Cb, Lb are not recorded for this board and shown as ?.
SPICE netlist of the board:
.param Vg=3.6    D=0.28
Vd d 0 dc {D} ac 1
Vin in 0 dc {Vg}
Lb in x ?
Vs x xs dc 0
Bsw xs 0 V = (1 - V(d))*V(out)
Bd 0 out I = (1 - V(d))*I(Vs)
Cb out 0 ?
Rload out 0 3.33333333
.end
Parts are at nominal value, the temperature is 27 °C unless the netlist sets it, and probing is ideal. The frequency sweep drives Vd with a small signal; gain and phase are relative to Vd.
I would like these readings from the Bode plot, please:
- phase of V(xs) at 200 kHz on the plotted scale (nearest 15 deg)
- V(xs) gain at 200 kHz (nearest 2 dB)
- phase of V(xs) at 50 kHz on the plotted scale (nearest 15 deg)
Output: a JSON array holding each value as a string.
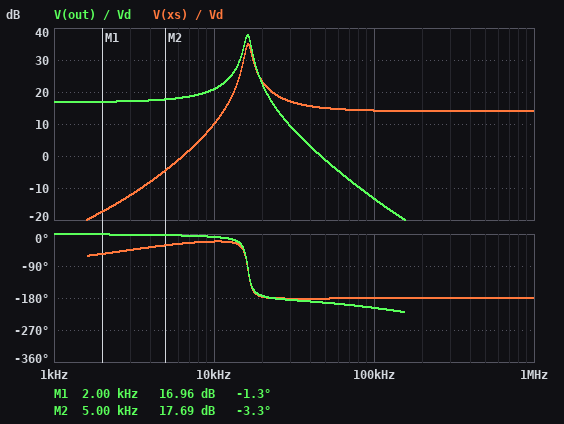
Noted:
["-180 deg", "14 dB", "-180 deg"]
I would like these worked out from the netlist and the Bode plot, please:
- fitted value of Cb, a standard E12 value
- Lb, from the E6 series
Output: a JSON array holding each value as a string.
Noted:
["33 µF", "1.5 µH"]
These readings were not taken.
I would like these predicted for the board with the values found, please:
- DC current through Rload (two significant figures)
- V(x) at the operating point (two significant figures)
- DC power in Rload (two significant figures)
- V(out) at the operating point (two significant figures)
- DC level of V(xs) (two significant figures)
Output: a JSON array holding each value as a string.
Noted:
["1.5 A", "3.6 V", "7.5 W", "5.0 V", "3.6 V"]
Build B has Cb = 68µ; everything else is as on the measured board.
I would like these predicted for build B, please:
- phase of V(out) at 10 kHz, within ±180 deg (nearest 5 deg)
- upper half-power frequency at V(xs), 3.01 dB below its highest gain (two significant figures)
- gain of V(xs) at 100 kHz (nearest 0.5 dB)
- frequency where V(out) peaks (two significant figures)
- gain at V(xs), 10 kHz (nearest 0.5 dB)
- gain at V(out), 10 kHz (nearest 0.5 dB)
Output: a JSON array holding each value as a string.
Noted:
["-15 deg", "12 kHz", "14.0 dB", "11 kHz", "24.5 dB", "29.5 dB"]
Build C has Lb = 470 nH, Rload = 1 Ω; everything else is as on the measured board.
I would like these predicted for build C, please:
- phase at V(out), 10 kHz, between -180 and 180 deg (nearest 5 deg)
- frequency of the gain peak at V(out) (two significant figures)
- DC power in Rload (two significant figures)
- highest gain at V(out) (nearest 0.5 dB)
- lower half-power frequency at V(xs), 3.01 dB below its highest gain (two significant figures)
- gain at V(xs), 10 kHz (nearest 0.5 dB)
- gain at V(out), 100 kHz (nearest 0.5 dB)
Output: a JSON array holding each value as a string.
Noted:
["-5 deg", "29 kHz", "25 W", "32.5 dB", "27 kHz", "-0.5 dB", "-2.5 dB"]
